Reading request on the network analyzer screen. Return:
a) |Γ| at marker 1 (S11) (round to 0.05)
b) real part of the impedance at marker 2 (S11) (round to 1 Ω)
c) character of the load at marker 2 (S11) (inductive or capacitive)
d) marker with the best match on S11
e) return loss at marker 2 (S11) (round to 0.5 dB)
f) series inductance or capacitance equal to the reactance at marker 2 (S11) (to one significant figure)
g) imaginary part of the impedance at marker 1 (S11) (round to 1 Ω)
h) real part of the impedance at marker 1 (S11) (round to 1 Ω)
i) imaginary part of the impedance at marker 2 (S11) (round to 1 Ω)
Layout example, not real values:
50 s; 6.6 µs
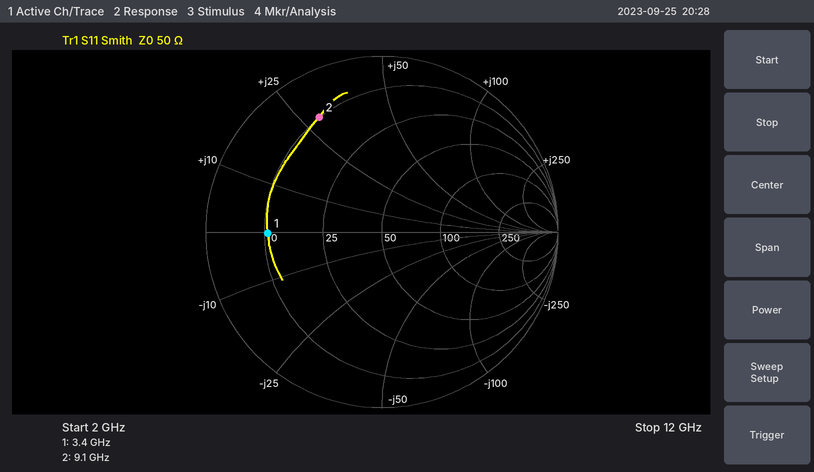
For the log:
0.65; 10 Ω; inductive; marker 1; 2.5 dB; 500 pH; 0 Ω; 11 Ω; +29 Ω
